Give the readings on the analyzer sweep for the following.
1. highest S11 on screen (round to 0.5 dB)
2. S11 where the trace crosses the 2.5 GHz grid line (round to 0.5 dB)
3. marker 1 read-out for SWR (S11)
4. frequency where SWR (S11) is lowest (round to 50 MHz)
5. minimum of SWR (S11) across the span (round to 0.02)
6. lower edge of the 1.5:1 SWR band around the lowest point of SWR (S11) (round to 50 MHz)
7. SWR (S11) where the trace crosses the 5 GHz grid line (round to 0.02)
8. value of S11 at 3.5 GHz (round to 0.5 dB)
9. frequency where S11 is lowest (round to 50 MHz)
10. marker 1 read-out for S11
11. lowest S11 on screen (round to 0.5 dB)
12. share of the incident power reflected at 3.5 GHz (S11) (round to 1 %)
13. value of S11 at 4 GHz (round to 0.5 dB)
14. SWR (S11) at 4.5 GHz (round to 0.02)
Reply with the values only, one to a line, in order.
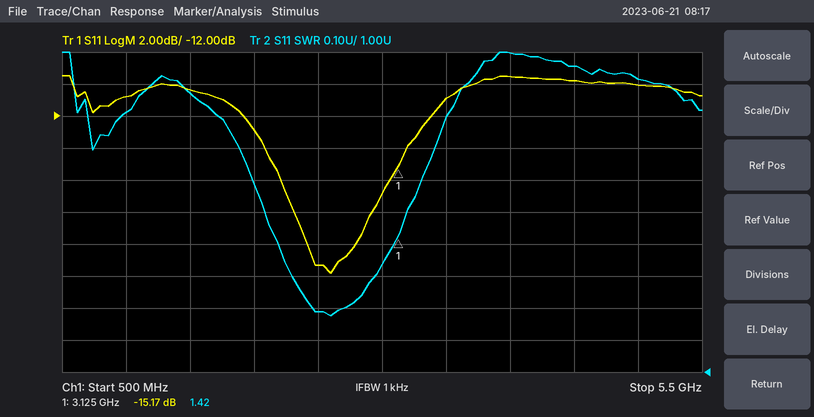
-9.5 dB
-21.5 dB
1.42
2.60 GHz
1.18
2.10 GHz
1.92
-11.0 dB
2.60 GHz
-15.17 dB
-22.0 dB
8 %
-9.5 dB
1.96
